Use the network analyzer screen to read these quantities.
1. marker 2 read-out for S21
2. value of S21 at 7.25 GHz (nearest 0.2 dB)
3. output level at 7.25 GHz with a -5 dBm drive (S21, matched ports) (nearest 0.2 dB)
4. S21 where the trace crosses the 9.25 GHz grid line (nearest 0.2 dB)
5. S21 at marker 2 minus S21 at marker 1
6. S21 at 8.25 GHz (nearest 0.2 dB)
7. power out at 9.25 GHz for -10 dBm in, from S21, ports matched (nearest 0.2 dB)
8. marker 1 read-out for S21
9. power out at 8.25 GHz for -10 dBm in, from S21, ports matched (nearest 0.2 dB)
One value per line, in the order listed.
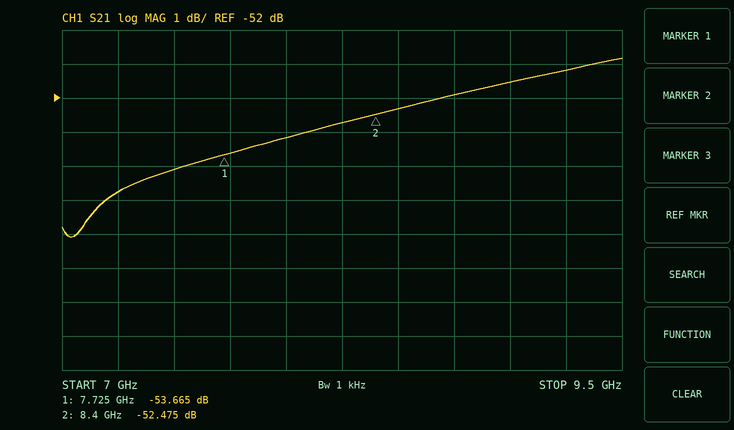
-52.475 dB
-54.8 dB
-59.8 dBm
-51.2 dB
1.190 dB
-52.8 dB
-61.2 dBm
-53.665 dB
-62.8 dBm
